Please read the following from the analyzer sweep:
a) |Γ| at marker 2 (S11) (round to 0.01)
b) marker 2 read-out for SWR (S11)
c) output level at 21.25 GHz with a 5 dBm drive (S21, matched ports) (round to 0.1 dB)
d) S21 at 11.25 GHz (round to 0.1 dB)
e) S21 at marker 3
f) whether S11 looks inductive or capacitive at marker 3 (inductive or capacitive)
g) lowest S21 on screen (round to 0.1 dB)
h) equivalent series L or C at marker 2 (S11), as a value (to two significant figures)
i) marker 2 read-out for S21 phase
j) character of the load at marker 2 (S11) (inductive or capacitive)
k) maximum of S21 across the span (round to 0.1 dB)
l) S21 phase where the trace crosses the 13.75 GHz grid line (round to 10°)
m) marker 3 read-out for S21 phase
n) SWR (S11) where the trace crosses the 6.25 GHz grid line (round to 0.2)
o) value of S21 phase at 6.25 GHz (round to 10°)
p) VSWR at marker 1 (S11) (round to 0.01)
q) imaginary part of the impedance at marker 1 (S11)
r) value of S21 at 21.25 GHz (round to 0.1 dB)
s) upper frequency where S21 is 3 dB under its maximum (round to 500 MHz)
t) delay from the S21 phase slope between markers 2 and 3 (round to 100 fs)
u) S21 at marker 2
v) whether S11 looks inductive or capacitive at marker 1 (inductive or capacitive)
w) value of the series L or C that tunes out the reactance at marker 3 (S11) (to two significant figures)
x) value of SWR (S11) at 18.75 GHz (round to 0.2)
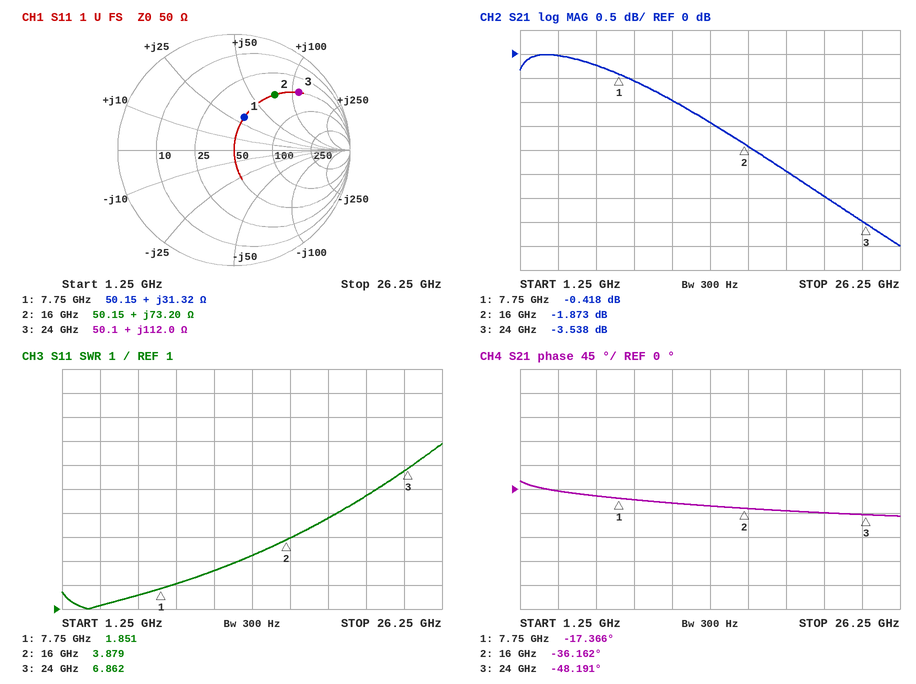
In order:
0.59
3.879
2.0 dBm
-1.0 dB
-3.538 dB
inductive
-4.0 dB
730 pH
-36.162°
inductive
0.0 dB
-30°
-48.191°
1.6
-10°
1.85
+31.32 Ω
-3.0 dB
21.5 GHz
4.2 ps
-1.873 dB
inductive
59 fF
4.8
